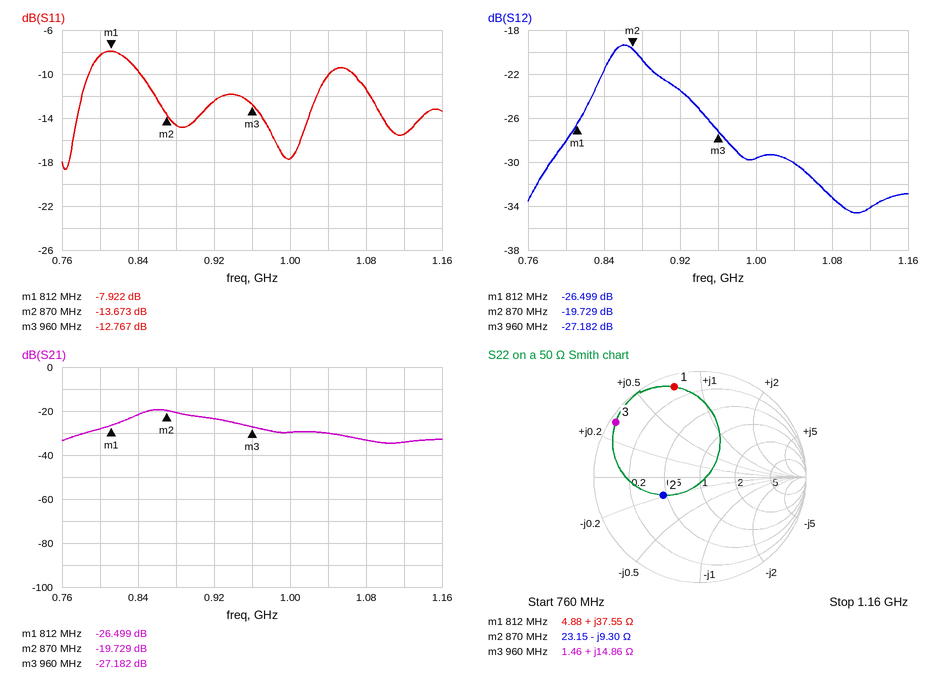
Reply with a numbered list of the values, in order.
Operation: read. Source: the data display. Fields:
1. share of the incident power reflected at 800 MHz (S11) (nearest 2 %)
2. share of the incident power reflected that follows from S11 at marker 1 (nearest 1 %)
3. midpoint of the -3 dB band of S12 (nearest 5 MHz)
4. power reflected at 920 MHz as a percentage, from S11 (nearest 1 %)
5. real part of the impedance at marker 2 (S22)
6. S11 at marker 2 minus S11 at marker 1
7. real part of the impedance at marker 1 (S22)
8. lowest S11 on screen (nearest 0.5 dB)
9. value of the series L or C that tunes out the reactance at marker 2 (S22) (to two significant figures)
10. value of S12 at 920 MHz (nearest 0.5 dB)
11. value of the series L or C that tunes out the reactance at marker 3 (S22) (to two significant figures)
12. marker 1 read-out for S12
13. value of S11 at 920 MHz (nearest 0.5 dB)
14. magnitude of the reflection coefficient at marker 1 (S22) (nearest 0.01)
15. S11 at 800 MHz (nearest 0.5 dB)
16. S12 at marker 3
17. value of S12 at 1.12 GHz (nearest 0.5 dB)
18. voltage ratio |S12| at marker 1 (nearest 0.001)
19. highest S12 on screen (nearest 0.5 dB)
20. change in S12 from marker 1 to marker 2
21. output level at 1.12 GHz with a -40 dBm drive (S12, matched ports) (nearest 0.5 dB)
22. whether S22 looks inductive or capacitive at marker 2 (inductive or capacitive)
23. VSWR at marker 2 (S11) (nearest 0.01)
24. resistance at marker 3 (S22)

1. 14 %
2. 16 %
3. 870 MHz
4. 6 %
5. 23.15 Ω
6. -5.751 dB
7. 4.88 Ω
8. -18.5 dB
9. 1.7 nH
10. -23.5 dB
11. 11 pF
12. -26.499 dB
13. -12.5 dB
14. 0.88
15. -8.5 dB
16. -27.182 dB
17. -34.0 dB
18. 0.047
19. -19.5 dB
20. 6.770 dB
21. -74.0 dBm
22. capacitive
23. 1.52
24. 1.46 Ω
